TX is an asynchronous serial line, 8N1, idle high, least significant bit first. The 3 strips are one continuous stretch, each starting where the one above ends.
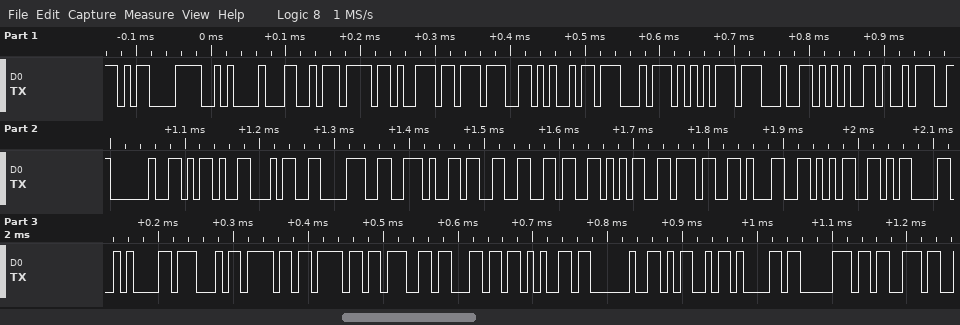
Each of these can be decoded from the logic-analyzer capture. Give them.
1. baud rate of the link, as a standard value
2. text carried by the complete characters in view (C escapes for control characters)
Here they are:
115200 baud
"\r\nLongitude: -48.365715\r\nGoogle Maps"
